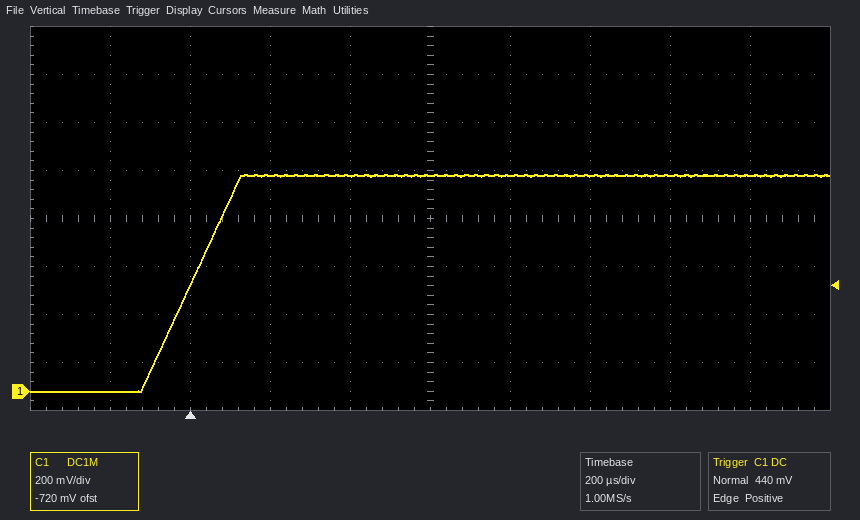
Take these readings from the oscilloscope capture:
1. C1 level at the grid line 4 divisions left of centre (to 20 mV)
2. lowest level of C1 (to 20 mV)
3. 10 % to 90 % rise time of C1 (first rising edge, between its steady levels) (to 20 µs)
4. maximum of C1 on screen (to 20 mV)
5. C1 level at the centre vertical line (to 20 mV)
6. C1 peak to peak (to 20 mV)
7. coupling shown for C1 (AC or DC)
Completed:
0 mV
0 mV
200 µs
900 mV
900 mV
900 mV
DC
